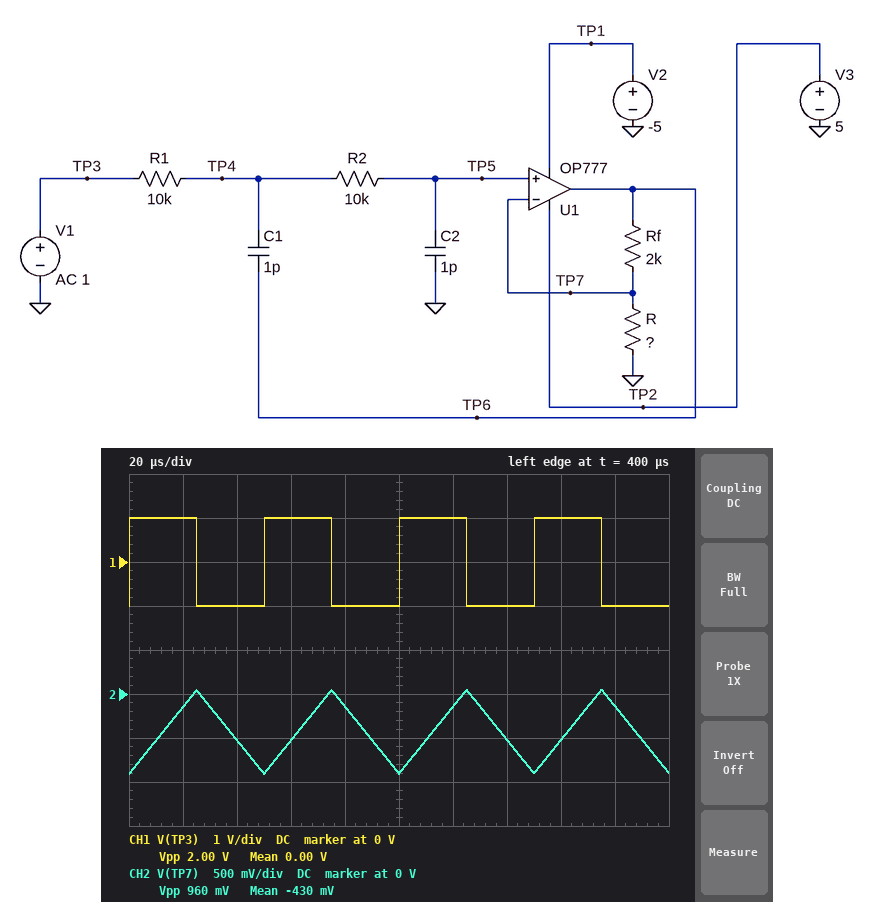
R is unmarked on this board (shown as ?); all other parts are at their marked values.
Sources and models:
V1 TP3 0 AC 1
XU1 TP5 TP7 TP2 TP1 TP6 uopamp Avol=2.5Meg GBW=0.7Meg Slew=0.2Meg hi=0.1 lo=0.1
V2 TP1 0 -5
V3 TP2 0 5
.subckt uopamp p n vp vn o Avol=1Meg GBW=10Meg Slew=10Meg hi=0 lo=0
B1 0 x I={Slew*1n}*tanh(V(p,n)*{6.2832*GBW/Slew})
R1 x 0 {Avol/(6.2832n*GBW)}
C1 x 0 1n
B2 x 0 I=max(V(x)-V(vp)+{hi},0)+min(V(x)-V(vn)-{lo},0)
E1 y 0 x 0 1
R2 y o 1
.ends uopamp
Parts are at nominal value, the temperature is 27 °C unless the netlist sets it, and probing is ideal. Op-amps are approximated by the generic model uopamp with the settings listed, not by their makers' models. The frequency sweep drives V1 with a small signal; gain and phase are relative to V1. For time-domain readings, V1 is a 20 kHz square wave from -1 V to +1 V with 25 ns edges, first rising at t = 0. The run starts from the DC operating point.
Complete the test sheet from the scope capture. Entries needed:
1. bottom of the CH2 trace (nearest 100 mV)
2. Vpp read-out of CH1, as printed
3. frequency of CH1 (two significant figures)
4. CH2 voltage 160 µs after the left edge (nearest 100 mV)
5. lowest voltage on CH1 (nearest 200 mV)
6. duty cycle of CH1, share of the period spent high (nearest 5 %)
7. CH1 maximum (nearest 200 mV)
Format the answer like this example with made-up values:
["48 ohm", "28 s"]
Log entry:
["-900 mV", "2.00 V", "20 kHz", "-500 mV", "-1.0 V", "50 %", "1.0 V"]
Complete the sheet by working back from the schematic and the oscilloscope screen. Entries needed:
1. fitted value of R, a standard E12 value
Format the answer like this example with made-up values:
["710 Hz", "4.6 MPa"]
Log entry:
["470 Ω"]
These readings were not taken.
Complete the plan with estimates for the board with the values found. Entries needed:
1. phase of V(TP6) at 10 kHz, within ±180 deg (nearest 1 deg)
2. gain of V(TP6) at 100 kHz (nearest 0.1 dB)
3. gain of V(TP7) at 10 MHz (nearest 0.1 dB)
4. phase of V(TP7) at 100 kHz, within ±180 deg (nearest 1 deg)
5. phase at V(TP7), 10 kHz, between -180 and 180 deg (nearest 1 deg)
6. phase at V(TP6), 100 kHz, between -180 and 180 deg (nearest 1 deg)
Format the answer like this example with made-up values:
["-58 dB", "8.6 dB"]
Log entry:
["-4 deg", "12.6 dB", "-43.4 dB", "-37 deg", "-4 deg", "-37 deg"]
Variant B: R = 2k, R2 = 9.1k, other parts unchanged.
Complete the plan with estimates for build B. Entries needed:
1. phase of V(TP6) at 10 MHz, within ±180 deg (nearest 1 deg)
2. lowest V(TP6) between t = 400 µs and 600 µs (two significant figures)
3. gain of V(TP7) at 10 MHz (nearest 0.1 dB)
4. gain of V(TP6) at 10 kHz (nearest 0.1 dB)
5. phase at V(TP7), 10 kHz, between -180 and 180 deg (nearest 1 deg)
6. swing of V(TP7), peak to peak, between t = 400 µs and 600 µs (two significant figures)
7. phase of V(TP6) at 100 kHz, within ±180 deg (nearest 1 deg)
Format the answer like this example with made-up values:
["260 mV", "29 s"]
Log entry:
["-160 deg", "-2.0 V", "-34.8 dB", "6.0 dB", "-2 deg", "2.0 V", "-16 deg"]
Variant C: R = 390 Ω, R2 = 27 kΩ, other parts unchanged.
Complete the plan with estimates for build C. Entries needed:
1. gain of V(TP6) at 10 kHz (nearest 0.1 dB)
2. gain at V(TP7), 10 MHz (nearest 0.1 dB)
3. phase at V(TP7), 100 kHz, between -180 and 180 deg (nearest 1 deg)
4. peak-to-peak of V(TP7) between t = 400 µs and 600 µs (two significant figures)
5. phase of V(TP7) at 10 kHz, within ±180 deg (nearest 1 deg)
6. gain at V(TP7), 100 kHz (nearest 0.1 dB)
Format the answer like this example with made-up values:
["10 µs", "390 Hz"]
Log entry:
["15.7 dB", "-48.3 dB", "-42 deg", "820 mV", "-5 deg", "-2.3 dB"]
